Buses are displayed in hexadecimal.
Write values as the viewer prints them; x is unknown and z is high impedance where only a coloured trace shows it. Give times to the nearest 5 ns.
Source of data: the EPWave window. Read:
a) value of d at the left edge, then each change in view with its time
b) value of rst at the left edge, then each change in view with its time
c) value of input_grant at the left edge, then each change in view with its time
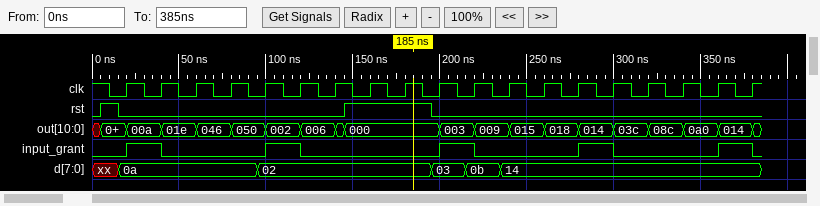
xx, 0a at 15 ns, 02 at 95 ns, 03 at 195 ns, 0b at 215 ns, 14 at 235 ns
0, 1 at 5 ns, 0 at 15 ns, 1 at 145 ns, 0 at 195 ns
0, 1 at 20 ns, 0 at 40 ns, 1 at 100 ns, 0 at 120 ns, 1 at 200 ns, 0 at 220 ns, 1 at 280 ns, 0 at 300 ns, 1 at 360 ns, 0 at 380 ns
